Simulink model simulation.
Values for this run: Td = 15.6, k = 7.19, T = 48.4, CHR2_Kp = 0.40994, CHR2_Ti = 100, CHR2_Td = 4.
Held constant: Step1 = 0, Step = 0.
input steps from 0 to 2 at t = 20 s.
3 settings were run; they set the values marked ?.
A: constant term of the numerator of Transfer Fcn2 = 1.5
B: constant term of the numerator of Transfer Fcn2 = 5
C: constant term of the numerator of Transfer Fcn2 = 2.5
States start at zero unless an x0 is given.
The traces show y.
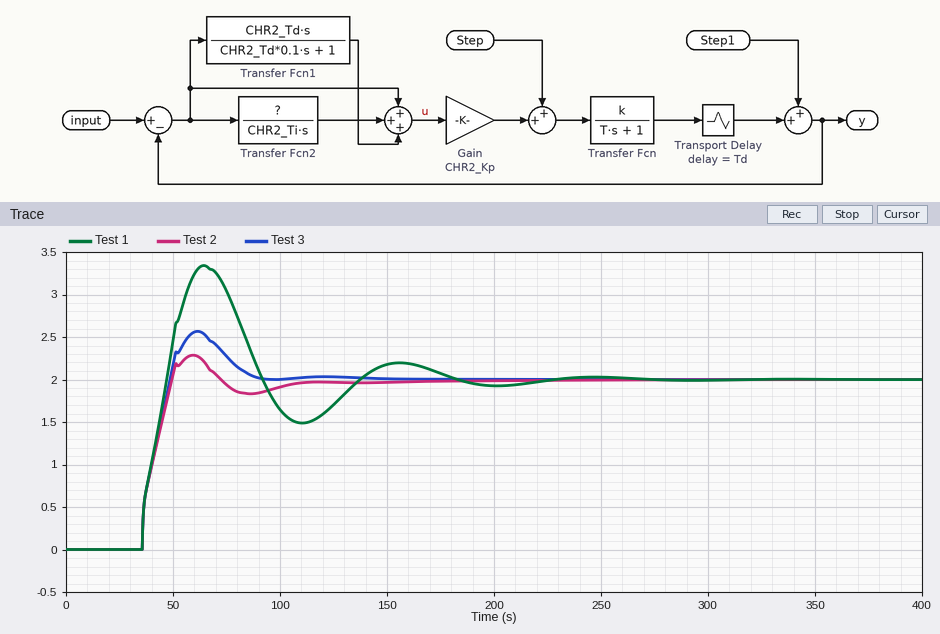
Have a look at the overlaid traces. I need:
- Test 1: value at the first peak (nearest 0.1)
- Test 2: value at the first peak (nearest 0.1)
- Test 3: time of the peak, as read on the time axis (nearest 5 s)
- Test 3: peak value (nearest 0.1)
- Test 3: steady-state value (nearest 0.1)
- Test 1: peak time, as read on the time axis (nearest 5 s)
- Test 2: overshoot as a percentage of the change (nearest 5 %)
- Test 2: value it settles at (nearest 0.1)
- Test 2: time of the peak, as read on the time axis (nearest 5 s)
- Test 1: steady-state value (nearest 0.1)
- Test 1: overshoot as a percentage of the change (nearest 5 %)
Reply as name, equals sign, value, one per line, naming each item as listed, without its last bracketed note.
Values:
Test 1: value at the first peak = 3.3
Test 2: value at the first peak = 2.3
Test 3: time of the peak, as read on the time axis = 60 s
Test 3: peak value = 2.6
Test 3: steady-state value = 2.0
Test 1: peak time, as read on the time axis = 65 s
Test 2: overshoot as a percentage of the change = 15 %
Test 2: value it settles at = 2.0
Test 2: time of the peak, as read on the time axis = 60 s
Test 1: steady-state value = 2.0
Test 1: overshoot as a percentage of the change = 65 %
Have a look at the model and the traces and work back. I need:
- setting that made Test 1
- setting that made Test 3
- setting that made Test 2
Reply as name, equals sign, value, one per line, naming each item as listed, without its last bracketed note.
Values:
setting that made Test 1 = B
setting that made Test 3 = C
setting that made Test 2 = A
